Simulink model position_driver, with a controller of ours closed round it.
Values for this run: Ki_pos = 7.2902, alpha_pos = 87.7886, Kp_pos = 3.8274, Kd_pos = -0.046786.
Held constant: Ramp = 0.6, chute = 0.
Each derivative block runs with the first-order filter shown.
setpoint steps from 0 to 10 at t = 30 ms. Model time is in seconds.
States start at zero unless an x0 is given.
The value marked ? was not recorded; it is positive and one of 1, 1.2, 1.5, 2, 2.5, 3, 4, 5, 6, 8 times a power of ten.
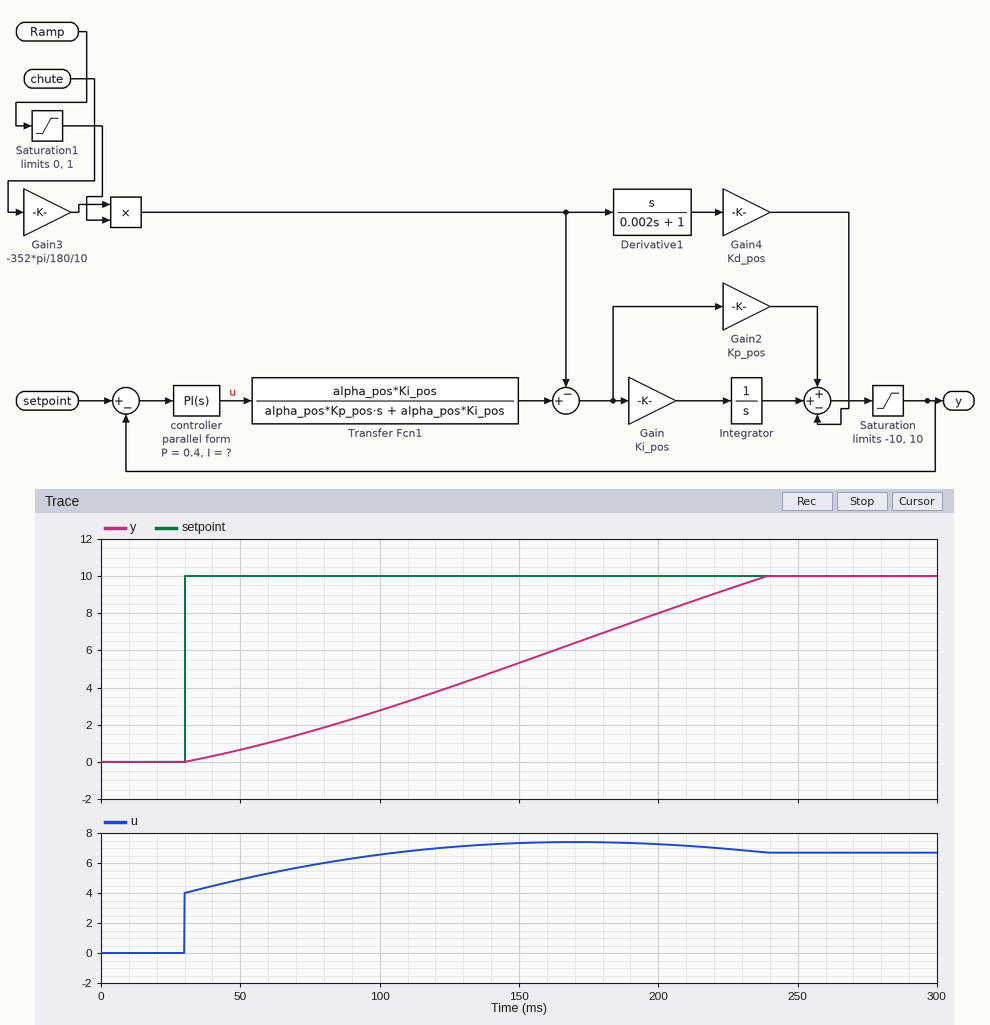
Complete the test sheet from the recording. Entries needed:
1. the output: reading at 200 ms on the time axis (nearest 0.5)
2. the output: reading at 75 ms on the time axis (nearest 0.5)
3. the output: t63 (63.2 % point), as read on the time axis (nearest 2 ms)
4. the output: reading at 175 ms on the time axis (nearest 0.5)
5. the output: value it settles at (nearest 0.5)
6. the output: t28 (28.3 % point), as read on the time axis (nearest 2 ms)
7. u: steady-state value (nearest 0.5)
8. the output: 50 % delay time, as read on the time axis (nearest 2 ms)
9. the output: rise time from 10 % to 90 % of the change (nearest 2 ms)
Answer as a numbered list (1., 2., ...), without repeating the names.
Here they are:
1. 8.0
2. 1.5
3. 168 ms
4. 6.5
5. 10.0
6. 102 ms
7. 6.5
8. 144 ms
9. 160 ms
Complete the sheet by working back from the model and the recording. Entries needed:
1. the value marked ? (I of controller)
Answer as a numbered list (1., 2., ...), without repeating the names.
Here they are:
1. 6
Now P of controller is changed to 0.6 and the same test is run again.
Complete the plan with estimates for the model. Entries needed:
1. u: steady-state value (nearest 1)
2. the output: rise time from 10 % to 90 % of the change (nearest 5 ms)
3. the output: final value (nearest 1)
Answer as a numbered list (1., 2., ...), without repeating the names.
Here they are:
1. 6
2. 155 ms
3. 10
